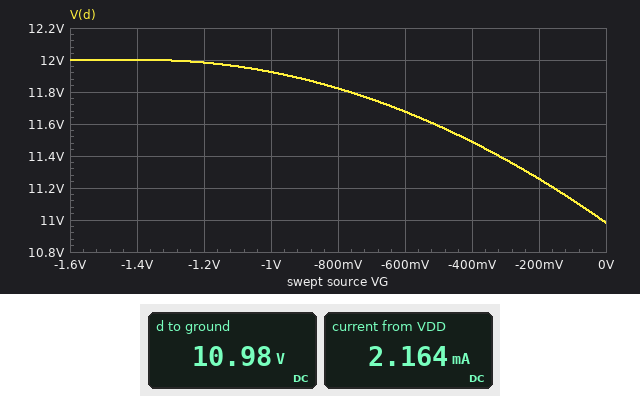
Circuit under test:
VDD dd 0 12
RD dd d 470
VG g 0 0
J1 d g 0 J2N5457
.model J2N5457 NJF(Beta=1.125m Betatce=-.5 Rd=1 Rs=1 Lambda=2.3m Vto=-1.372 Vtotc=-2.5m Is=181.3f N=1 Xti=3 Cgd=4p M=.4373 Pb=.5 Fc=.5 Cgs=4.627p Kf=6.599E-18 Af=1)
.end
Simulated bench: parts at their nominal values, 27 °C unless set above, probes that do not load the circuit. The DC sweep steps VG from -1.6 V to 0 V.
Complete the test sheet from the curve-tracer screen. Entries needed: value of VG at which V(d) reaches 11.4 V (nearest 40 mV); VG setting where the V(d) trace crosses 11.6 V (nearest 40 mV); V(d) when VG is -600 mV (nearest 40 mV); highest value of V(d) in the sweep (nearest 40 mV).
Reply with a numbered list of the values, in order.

1. -320 mV
2. -520 mV
3. 11.68 V
4. 12.00 V
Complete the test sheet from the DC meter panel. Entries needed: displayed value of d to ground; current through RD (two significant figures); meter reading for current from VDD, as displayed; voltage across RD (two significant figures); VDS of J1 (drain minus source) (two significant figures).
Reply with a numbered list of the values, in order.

1. 10.98 V
2. 2.2 mA
3. 2.164 mA
4. 1.0 V
5. 11 V
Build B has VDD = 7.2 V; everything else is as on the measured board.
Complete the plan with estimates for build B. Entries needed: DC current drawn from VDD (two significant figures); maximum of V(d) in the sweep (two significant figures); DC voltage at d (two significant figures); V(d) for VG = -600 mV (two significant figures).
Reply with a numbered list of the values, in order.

1. 2.1 mA
2. 7.2 V
3. 6.2 V
4. 6.9 V
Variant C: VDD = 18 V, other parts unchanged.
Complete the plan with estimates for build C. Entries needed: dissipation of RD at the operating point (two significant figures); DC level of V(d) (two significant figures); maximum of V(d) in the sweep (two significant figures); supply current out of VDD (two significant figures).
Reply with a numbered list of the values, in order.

1. 2.3 mW
2. 17 V
3. 18 V
4. 2.2 mA
